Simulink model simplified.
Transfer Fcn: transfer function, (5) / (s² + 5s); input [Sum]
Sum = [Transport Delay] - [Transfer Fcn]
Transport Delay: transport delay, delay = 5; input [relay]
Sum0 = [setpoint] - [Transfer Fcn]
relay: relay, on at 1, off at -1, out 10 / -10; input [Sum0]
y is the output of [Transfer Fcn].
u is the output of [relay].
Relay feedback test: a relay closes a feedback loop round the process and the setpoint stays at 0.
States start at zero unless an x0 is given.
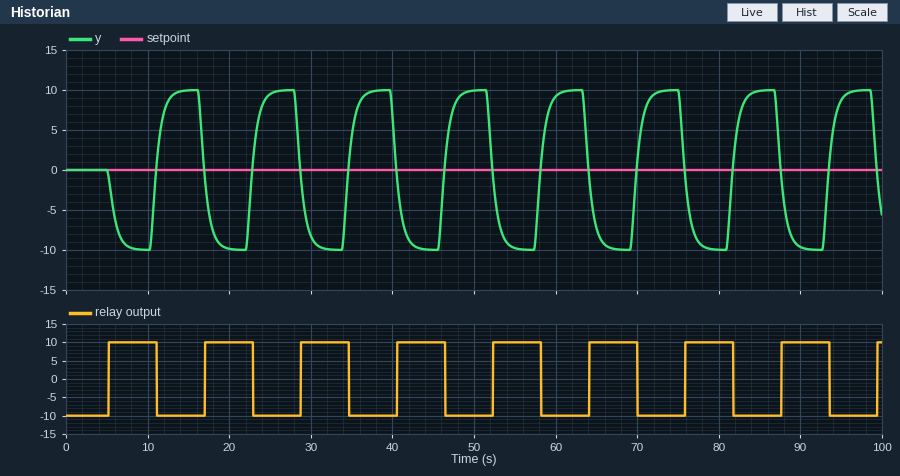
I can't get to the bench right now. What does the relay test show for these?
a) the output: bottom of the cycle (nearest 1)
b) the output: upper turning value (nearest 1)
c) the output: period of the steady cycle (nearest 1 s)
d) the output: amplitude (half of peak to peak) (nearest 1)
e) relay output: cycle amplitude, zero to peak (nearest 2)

-10
10
12 s
10
10
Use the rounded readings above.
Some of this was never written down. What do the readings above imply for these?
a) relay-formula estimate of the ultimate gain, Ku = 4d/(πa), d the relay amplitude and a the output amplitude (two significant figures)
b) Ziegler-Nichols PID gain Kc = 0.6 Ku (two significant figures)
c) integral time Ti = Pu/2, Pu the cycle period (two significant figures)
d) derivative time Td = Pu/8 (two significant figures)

1.3
0.78
6.0 s
1.5 s
